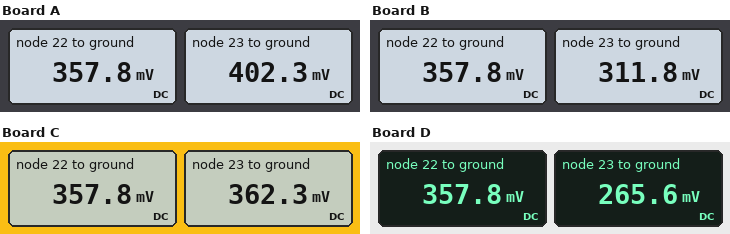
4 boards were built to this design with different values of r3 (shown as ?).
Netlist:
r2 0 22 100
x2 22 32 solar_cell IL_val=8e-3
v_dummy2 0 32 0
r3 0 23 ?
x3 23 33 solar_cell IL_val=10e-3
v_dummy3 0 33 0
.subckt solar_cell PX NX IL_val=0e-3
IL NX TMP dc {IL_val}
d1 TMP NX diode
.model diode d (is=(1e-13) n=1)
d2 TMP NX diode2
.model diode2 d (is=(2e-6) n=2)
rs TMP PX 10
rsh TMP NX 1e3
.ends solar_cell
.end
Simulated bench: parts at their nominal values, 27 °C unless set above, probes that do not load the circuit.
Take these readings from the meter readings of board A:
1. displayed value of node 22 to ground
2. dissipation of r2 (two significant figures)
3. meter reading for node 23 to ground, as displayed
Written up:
357.8 mV
1.3 mW
402.3 mV
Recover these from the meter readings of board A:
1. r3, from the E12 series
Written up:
180 Ω
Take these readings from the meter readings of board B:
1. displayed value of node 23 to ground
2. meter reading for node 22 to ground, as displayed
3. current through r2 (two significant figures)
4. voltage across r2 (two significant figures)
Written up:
311.8 mV
357.8 mV
3.6 mA
360 mV
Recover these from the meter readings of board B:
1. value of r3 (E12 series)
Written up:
47 Ω
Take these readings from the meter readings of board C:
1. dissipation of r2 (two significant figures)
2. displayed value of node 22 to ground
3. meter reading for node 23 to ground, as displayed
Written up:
1.3 mW
357.8 mV
362.3 mV
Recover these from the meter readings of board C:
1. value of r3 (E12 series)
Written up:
82 Ω
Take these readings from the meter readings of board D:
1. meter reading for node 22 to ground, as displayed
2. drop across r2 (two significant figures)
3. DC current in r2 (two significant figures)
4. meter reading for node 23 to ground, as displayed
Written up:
357.8 mV
360 mV
3.6 mA
265.6 mV
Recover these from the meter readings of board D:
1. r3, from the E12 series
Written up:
33 Ω
